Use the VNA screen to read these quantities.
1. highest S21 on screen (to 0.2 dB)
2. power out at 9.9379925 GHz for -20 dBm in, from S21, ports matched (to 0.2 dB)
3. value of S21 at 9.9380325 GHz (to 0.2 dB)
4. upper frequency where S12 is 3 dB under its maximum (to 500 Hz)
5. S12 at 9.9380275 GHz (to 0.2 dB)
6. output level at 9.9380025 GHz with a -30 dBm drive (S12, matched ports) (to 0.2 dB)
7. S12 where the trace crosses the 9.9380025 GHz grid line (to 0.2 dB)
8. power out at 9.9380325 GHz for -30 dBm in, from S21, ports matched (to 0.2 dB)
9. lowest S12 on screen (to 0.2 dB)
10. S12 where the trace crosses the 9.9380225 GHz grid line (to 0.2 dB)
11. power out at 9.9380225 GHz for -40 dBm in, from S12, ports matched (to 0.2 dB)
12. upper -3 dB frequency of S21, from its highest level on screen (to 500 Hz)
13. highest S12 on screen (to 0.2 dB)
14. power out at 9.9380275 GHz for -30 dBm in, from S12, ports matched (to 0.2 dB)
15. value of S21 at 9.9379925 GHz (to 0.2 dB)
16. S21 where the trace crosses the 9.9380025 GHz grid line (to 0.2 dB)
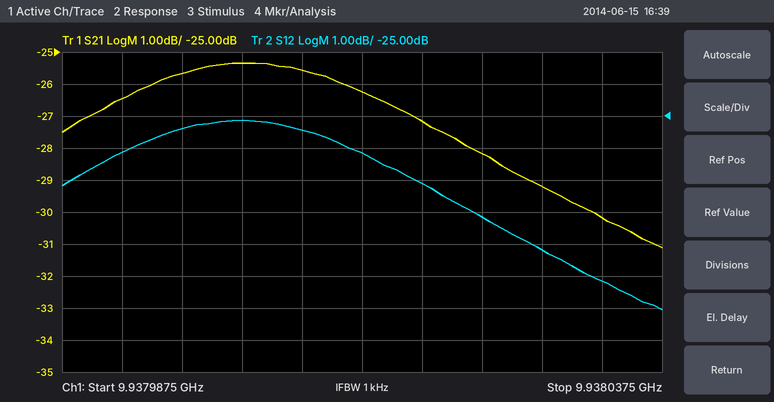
-25.4 dB
-46.4 dBm
-30.2 dB
9.9380225 GHz
-29.2 dB
-55.2 dBm
-25.2 dB
-60.2 dBm
-31.0 dB
-28.2 dB
-68.2 dBm
9.9380235 GHz
-25.2 dB
-59.2 dBm
-26.4 dB
-25.4 dB
